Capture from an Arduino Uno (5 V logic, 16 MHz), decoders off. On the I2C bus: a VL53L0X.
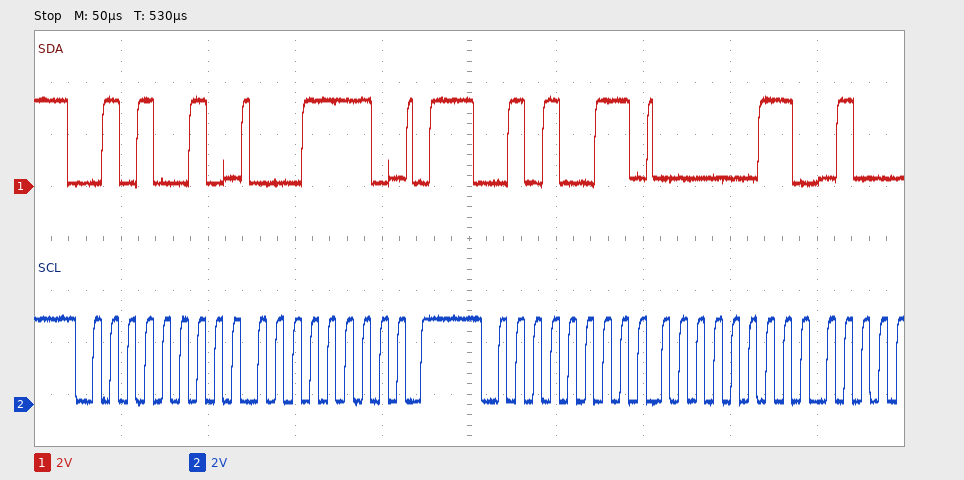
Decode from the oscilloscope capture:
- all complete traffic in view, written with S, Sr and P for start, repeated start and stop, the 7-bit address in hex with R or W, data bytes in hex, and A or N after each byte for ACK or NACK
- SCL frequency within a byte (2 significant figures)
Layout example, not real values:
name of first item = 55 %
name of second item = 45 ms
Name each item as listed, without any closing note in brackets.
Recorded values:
all complete traffic in view, written with S, Sr and P for start, repeated start and stop, the 7-bit address in hex with R or W, data bytes in hex, and A or N after each byte for ACK or NACK = S 29W A 1E A P S 29R A 03 A
SCL frequency within a byte = 100 kHz
